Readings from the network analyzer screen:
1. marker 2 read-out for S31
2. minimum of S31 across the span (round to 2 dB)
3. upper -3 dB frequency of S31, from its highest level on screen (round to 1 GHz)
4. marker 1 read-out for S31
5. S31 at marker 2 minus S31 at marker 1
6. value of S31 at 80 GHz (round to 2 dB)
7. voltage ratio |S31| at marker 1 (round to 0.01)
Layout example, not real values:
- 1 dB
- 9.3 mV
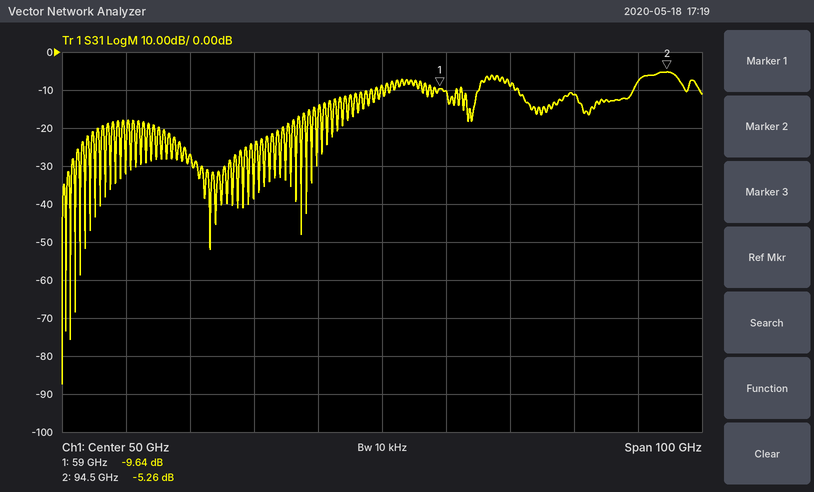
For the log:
- -5.26 dB
- -88 dB
- 97 GHz
- -9.64 dB
- 4.38 dB
- -12 dB
- 0.33
